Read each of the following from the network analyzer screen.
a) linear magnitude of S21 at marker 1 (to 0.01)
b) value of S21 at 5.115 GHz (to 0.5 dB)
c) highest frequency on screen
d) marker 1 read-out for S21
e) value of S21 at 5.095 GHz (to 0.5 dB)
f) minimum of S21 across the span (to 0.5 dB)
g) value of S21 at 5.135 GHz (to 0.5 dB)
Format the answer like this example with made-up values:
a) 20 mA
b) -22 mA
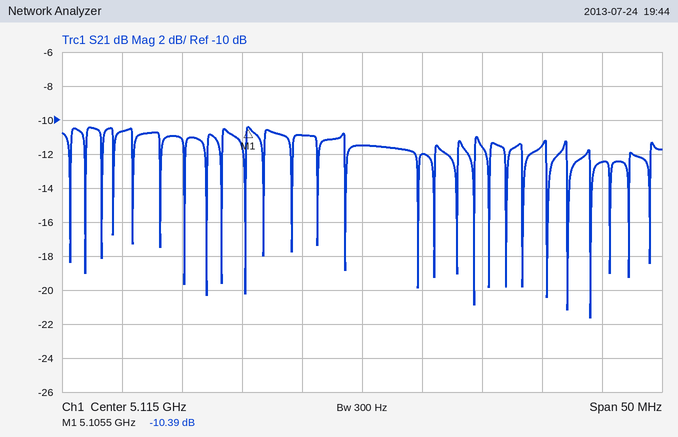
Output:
a) 0.30
b) -11.5 dB
c) 5.14 GHz
d) -10.39 dB
e) -10.5 dB
f) -21.5 dB
g) -12.5 dB
